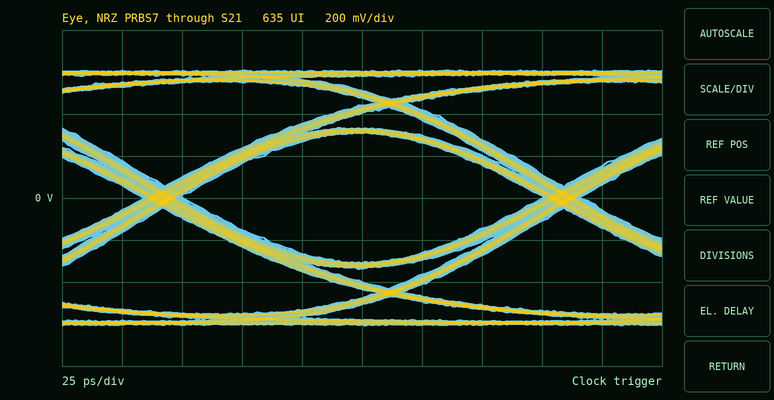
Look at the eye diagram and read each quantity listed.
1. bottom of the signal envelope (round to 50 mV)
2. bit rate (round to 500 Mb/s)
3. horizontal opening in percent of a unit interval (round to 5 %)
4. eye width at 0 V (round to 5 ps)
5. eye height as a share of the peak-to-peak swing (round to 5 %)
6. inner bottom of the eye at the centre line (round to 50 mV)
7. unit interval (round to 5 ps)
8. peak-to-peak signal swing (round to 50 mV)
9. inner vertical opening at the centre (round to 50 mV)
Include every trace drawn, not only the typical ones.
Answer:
-600 mV
6.0 Gb/s
90 %
150 ps
50 %
-300 mV
165 ps
1.20 V
600 mV
